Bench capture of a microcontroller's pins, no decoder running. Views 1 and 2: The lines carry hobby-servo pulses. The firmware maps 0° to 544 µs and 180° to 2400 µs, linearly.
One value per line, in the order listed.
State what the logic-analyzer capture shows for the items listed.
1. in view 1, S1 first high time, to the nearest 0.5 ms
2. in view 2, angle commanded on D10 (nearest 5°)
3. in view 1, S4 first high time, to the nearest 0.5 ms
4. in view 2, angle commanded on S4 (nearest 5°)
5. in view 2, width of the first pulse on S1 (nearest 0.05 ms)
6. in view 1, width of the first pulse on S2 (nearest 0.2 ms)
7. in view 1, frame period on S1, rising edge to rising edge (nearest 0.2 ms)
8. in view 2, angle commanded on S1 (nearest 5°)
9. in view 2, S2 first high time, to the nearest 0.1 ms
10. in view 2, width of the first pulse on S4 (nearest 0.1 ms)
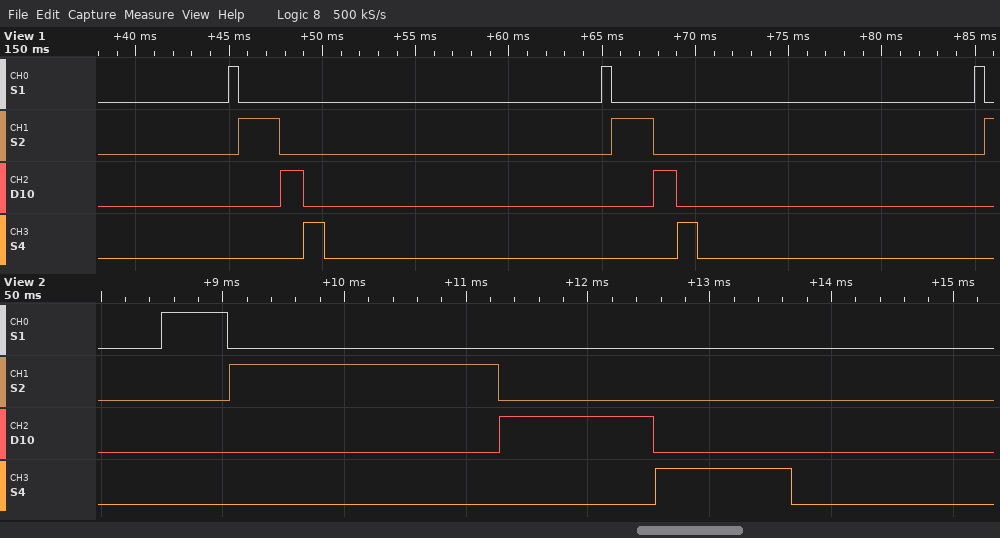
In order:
0.5 ms
70°
1.0 ms
55°
0.55 ms
2.2 ms
20.0 ms
0°
2.2 ms
1.1 ms
